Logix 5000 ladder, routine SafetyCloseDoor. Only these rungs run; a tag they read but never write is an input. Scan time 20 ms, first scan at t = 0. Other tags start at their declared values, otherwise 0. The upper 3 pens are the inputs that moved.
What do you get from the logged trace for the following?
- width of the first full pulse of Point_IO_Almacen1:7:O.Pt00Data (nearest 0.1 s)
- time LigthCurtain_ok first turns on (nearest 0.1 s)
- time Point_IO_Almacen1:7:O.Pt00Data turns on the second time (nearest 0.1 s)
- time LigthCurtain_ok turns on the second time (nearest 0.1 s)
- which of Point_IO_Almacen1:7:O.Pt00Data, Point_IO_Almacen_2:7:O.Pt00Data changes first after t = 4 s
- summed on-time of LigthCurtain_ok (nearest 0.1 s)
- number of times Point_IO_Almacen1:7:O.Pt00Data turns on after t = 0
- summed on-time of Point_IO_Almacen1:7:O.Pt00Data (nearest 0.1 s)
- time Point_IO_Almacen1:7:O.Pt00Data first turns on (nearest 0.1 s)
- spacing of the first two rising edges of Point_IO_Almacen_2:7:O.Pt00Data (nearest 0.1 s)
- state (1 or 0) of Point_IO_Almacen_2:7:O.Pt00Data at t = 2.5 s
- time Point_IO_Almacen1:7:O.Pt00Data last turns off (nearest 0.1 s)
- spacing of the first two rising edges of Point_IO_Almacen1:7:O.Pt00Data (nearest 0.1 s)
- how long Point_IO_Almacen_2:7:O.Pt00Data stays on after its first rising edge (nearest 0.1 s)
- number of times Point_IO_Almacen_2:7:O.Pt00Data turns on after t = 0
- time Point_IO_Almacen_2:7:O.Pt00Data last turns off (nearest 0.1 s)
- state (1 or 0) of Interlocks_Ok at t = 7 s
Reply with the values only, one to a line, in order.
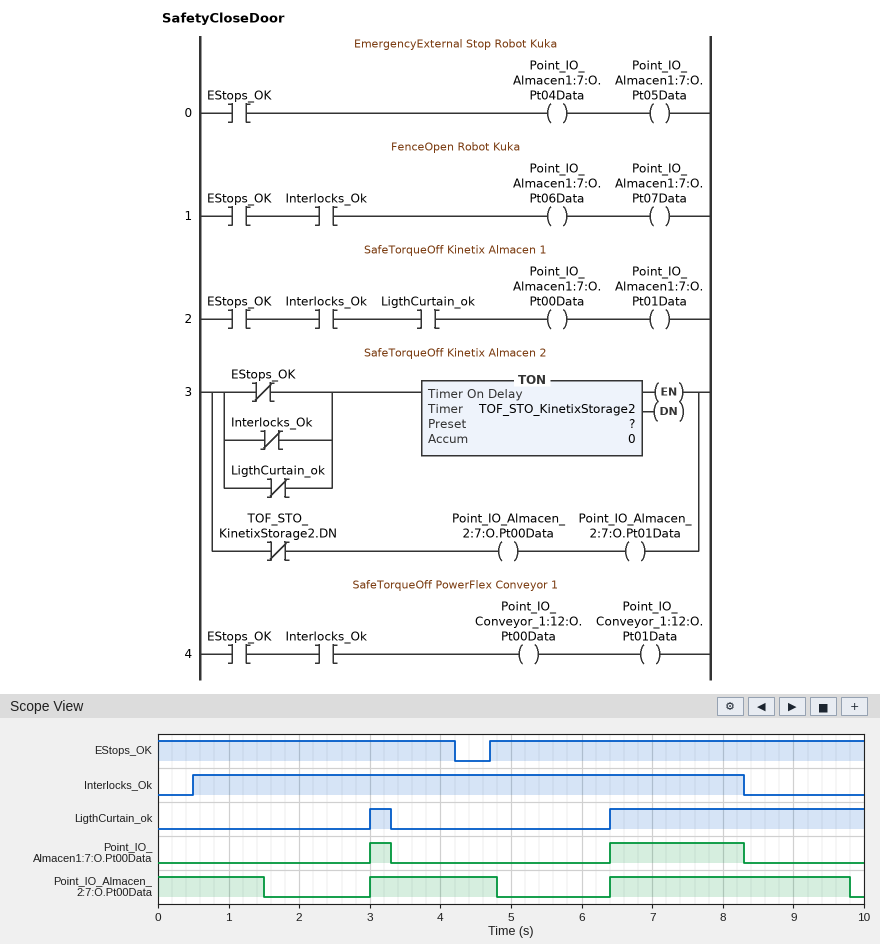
0.3 s
3.0 s
6.4 s
6.4 s
Point_IO_Almacen_2:7:O.Pt00Data
3.9 s
2
2.2 s
3.0 s
3.4 s
0
8.3 s
3.4 s
1.8 s
2
9.8 s
1
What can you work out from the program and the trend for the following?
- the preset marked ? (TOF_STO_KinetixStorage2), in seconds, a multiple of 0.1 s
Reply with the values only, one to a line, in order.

1.5 s
